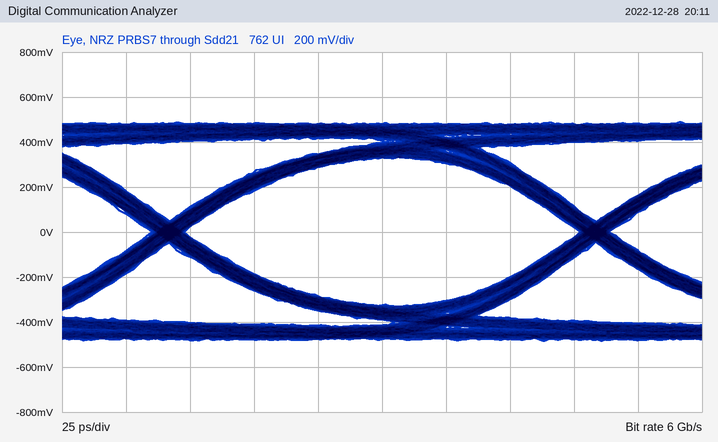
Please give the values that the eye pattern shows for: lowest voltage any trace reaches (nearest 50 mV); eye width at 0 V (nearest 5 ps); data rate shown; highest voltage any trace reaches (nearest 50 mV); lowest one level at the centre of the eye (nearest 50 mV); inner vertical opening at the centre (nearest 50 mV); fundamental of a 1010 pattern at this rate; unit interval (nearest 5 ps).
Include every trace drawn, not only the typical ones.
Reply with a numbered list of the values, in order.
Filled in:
1. -500 mV
2. 155 ps
3. 6 Gb/s
4. 500 mV
5. 350 mV
6. 650 mV
7. 3 GHz
8. 165 ps
